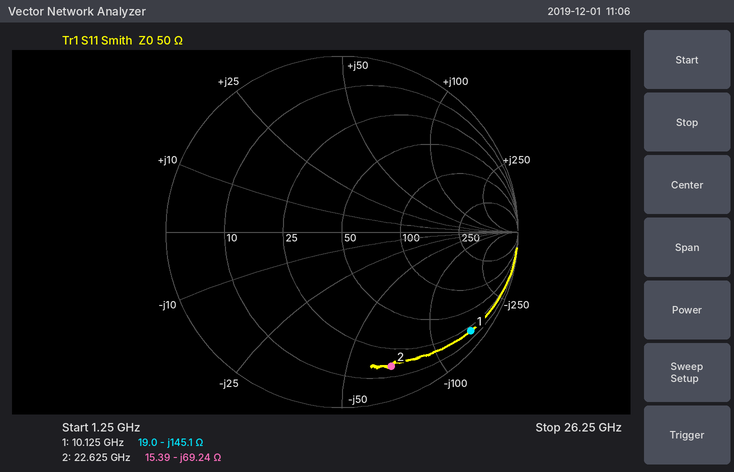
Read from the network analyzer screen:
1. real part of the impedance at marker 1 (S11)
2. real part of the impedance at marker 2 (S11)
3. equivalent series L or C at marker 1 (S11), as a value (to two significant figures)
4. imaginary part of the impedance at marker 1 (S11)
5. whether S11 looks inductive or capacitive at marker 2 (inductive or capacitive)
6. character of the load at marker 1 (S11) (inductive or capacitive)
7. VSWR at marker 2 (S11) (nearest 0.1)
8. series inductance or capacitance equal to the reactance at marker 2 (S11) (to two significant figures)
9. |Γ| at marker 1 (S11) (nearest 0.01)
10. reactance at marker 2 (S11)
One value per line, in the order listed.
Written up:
19.0 Ω
15.39 Ω
110 fF
-145.1 Ω
capacitive
capacitive
9.7
100 fF
0.92
-69.24 Ω
